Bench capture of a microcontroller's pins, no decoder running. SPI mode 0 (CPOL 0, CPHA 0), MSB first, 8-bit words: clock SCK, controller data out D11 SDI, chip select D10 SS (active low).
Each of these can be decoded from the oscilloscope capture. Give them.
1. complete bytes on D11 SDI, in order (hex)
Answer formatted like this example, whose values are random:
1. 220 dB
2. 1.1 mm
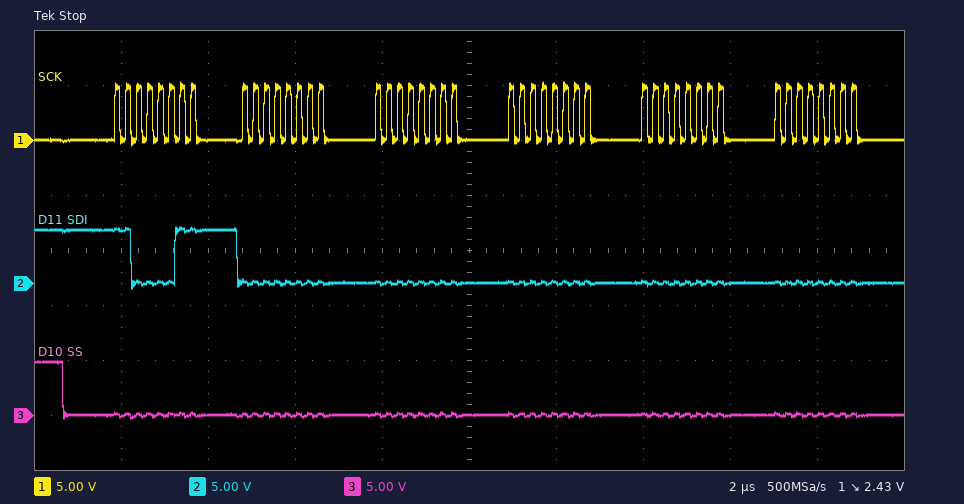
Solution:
1. C3 00 00 00 00 00
